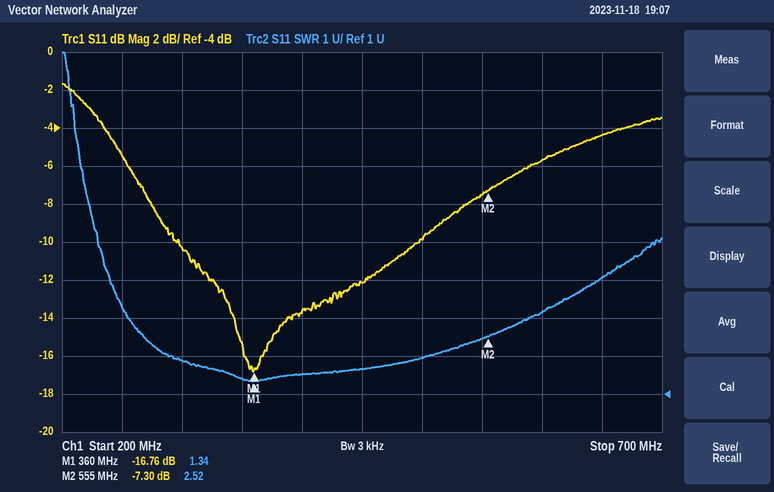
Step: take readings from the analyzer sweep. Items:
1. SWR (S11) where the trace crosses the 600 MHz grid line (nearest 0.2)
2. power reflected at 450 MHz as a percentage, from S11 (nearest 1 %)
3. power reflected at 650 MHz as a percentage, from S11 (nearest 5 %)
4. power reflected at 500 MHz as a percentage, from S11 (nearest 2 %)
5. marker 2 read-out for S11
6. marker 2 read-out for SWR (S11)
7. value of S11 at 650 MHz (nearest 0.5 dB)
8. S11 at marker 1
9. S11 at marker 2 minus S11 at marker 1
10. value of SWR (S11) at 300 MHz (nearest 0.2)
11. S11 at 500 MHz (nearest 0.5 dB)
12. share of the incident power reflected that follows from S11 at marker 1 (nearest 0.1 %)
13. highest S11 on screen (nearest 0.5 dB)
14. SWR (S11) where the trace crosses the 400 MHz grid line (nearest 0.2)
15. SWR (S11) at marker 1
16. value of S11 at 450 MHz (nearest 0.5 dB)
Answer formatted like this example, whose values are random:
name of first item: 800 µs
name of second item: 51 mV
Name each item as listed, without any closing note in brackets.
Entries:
SWR (S11) where the trace crosses the 600 MHz grid line: 3.2
power reflected at 450 MHz as a percentage, from S11: 6 %
power reflected at 650 MHz as a percentage, from S11: 35 %
power reflected at 500 MHz as a percentage, from S11: 10 %
marker 2 read-out for S11: -7.30 dB
marker 2 read-out for SWR: 2.52
value of S11 at 650 MHz: -4.5 dB
S11 at marker 1: -16.76 dB
S11 at marker 2 minus S11 at marker 1: 9.46 dB
value of SWR (S11) at 300 MHz: 1.8
S11 at 500 MHz: -10.0 dB
share of the incident power reflected that follows from S11 at marker 1: 2.1 %
highest S11 on screen: -1.5 dB
SWR (S11) where the trace crosses the 400 MHz grid line: 1.6
SWR (S11) at marker 1: 1.34
value of S11 at 450 MHz: -12.0 dB
